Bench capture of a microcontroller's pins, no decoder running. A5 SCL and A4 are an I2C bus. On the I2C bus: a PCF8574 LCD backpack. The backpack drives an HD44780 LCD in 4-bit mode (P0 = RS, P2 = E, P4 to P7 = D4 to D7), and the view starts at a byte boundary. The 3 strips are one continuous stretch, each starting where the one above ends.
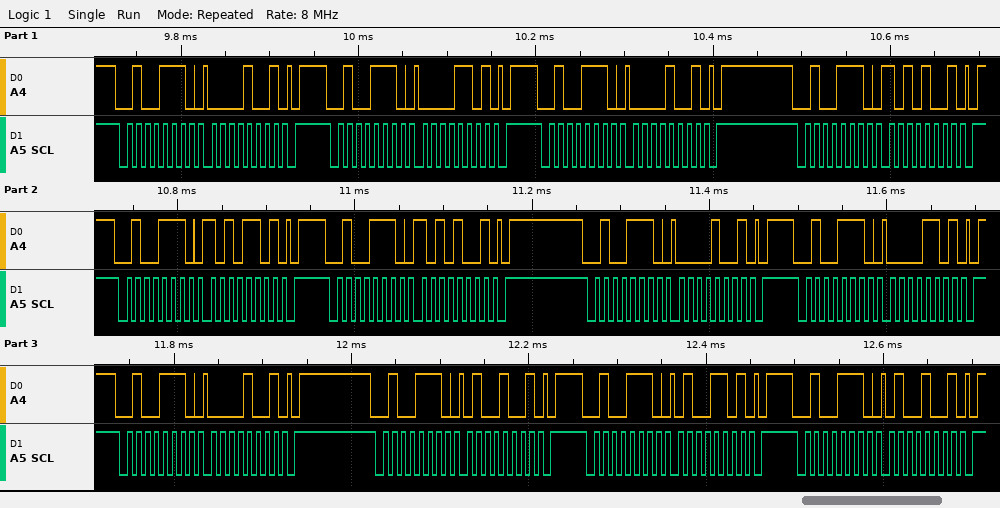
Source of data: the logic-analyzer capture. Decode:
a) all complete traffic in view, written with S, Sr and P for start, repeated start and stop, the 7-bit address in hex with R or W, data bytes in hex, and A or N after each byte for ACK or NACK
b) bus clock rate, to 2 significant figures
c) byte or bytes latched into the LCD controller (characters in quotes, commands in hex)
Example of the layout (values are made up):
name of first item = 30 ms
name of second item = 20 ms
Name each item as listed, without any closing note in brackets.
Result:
all complete traffic in view, written with S, Sr and P for start, repeated start and stop, the 7-bit address in hex with R or W, data bytes in hex, and A or N after each byte for ACK or NACK = S 27W A 09 A P S 27W A 0D A P S 27W A 09 A P S 27W A A9 A P S 27W A AD A P S 27W A A9 A P S 27W A 09 A P S 27W A 0D A P S 27W A 09 A P S 27W A 49 A P S 27W A 4D A P S 27W A 49 A P
bus clock rate, to 2 significant figures = 100 kHz
byte or bytes latched into the LCD controller = data 0x0A data 0x04
